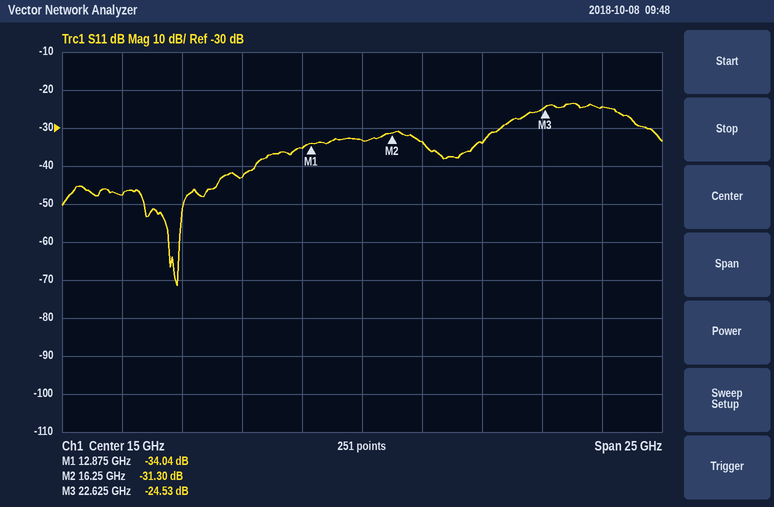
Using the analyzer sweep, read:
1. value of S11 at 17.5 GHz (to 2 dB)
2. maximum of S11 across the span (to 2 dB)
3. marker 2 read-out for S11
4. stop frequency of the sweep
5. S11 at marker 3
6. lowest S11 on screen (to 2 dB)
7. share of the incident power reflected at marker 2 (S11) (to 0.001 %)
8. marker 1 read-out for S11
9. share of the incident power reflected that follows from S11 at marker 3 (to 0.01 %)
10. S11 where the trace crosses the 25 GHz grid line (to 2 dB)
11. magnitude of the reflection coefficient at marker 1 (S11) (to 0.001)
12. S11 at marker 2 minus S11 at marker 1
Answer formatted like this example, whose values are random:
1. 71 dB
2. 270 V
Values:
1. -34 dB
2. -24 dB
3. -31.30 dB
4. 27.5 GHz
5. -24.53 dB
6. -72 dB
7. 0.074 %
8. -34.04 dB
9. 0.35 %
10. -24 dB
11. 0.020
12. 2.74 dB
